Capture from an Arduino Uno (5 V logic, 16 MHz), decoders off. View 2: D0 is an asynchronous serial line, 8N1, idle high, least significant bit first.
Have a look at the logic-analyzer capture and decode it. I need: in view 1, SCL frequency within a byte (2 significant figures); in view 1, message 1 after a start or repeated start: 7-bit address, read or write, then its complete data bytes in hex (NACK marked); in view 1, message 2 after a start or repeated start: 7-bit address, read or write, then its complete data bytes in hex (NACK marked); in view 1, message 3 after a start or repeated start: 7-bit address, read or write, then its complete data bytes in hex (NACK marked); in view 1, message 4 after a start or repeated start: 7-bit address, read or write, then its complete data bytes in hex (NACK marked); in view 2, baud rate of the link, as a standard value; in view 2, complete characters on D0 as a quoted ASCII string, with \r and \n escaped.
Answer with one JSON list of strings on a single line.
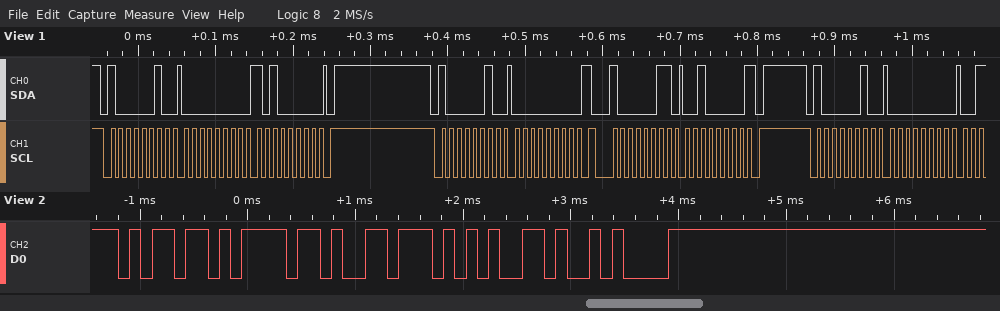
["100 kHz", "0x41 write: 00 A0", "0x41 write: 00", "0x41 read: 20 NACK", "0x41 write: 00", "9600 baud", "\"move\\n\""]
